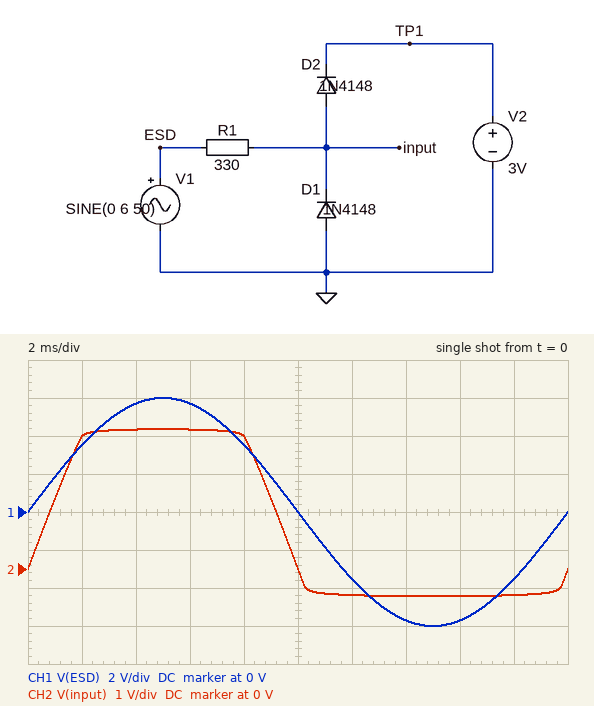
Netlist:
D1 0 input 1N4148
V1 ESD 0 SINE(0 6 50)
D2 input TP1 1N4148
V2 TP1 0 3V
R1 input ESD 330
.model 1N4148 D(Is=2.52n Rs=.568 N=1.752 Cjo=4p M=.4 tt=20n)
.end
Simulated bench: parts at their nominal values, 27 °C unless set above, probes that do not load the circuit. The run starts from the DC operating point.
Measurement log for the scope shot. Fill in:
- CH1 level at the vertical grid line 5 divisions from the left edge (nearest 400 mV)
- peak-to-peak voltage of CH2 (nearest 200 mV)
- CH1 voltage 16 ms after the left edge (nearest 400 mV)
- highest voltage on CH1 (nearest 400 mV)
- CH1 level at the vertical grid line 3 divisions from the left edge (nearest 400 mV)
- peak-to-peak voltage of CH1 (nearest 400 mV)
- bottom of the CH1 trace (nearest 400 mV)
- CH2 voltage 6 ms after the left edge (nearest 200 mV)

0 V
4.4 V
-5.6 V
6.0 V
5.6 V
12.0 V
-6.0 V
3.6 V
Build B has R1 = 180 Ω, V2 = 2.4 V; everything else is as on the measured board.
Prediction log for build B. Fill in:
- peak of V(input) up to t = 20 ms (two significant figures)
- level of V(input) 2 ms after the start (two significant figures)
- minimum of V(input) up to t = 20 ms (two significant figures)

3.1 V
3.0 V
-750 mV
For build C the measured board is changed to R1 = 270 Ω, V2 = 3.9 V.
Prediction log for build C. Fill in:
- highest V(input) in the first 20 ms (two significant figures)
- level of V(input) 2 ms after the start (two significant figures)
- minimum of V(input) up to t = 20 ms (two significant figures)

4.6 V
3.5 V
-730 mV
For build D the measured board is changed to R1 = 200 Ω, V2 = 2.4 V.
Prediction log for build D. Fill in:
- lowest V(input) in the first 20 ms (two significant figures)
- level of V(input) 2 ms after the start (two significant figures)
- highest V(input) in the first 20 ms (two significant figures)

-750 mV
3.0 V
3.1 V
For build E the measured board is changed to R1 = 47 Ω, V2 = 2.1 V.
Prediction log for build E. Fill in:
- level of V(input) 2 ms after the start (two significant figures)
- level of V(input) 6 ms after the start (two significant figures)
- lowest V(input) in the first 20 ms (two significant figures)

2.8 V
2.9 V
-860 mV
